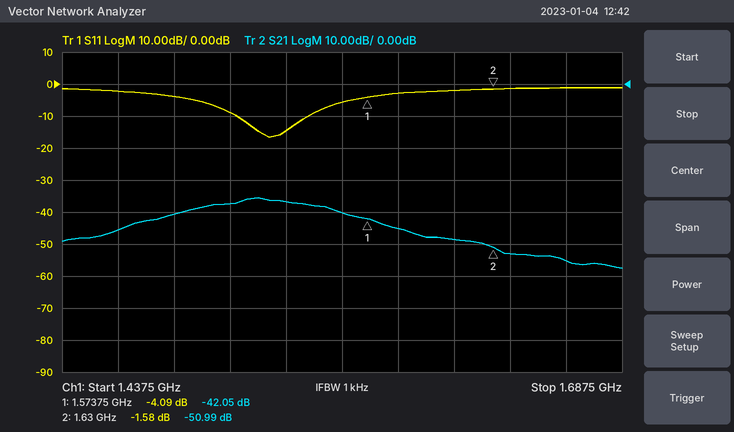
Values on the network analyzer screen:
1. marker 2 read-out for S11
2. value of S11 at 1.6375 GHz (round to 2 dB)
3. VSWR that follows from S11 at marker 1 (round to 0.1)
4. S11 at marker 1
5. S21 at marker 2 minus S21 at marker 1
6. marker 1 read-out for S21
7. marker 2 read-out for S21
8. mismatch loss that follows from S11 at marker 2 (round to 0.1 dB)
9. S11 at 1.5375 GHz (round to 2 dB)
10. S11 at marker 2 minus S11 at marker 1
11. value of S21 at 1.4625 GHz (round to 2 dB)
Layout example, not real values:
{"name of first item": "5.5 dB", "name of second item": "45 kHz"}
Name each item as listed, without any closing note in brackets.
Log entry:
{"marker 2 read-out for S11": "-1.58 dB", "value of S11 at 1.6375 GHz": "-2 dB", "VSWR that follows from S11 at marker 1": "4.3", "S11 at marker 1": "-4.09 dB", "S21 at marker 2 minus S21 at marker 1": "-8.94 dB", "marker 1 read-out for S21": "-42.05 dB", "marker 2 read-out for S21": "-50.99 dB", "mismatch loss that follows from S11 at marker 2": "5.2 dB", "S11 at 1.5375 GHz": "-14 dB", "S11 at marker 2 minus S11 at marker 1": "2.51 dB", "value of S21 at 1.4625 GHz": "-46 dB"}
